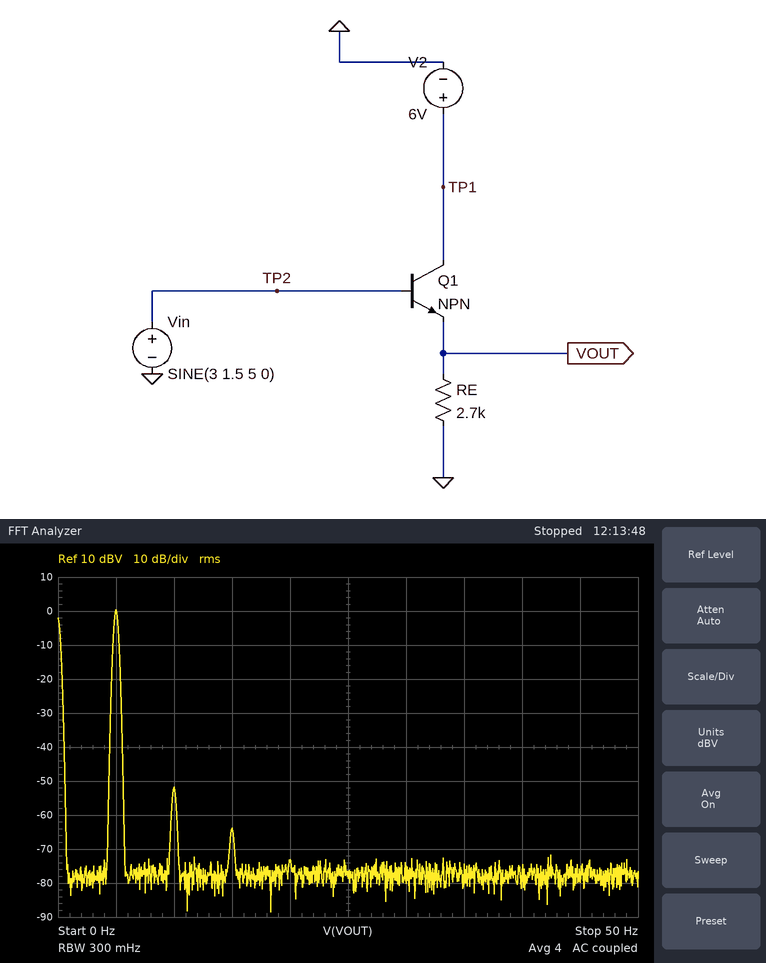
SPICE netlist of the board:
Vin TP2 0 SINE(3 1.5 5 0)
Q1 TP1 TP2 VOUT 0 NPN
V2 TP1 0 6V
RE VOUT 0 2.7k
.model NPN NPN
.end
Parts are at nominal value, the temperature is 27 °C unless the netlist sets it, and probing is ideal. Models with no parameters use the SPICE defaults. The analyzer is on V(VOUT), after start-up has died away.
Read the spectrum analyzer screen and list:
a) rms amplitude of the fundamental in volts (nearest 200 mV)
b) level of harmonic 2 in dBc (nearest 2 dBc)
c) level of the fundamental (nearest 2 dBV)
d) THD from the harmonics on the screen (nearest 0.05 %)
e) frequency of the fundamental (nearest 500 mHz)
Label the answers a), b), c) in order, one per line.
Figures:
a) 1.0 V
b) -52 dBc
c) 0 dBV
d) 0.25 %
e) 5.0 Hz
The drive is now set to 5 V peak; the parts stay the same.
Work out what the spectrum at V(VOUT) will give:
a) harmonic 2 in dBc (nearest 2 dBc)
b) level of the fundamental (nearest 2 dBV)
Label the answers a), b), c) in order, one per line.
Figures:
a) -18 dBc
b) 8 dBV
